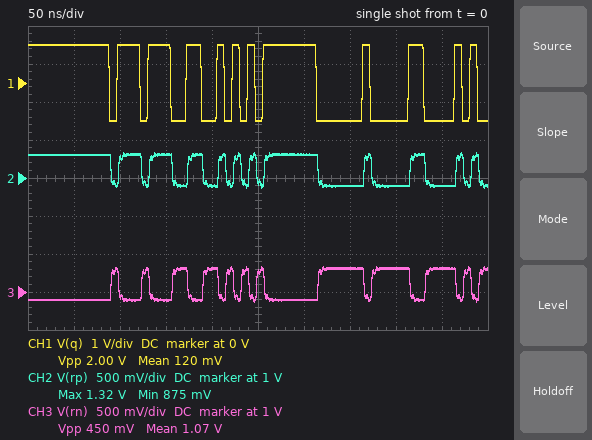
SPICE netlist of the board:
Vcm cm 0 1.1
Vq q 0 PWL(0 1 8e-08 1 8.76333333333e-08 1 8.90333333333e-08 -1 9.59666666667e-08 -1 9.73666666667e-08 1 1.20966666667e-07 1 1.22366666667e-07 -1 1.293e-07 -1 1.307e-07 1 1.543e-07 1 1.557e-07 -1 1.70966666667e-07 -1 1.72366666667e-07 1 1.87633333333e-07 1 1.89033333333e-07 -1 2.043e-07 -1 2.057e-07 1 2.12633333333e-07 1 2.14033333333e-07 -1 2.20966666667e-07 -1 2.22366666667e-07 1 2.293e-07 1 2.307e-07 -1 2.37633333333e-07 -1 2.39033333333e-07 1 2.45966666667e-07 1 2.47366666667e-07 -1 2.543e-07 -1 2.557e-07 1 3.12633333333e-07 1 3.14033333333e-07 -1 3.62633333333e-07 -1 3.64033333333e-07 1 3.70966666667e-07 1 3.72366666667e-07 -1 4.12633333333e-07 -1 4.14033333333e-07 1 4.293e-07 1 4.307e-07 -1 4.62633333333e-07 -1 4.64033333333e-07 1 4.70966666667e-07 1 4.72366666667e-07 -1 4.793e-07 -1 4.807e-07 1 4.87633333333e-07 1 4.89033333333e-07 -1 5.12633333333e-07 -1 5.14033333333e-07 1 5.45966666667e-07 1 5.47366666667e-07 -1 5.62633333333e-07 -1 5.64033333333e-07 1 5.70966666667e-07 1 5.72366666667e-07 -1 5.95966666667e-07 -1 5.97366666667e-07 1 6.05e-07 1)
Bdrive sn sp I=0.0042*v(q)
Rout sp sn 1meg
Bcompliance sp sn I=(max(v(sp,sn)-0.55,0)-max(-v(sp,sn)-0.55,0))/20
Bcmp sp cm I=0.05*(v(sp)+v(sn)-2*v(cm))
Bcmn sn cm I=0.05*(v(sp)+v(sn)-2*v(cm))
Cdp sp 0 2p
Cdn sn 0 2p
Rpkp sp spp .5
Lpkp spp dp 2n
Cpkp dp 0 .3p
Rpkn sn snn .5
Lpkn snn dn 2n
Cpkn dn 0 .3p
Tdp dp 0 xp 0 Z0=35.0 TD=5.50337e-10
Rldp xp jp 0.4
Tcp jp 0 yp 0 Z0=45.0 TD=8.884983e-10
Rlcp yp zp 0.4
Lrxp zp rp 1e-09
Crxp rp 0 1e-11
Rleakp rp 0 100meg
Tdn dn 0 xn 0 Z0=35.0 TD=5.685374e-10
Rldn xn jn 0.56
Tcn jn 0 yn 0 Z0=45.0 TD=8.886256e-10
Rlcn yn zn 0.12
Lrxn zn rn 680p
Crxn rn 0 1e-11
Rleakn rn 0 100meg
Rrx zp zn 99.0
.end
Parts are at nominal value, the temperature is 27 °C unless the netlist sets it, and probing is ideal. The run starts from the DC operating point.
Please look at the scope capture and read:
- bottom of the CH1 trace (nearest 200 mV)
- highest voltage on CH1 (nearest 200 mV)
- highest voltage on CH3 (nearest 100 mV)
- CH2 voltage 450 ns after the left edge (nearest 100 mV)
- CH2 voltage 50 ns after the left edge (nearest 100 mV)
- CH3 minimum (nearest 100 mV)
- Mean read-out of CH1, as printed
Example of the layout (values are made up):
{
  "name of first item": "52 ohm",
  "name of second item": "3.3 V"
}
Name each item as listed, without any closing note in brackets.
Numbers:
{
  "bottom of the CH1 trace": "-1.0 V",
  "highest voltage on CH1": "1.0 V",
  "highest voltage on CH3": "1.3 V",
  "CH2 voltage 450 ns after the left edge": "900 mV",
  "CH2 voltage 50 ns after the left edge": "1.3 V",
  "CH3 minimum": "900 mV",
  "Mean read-out of CH1, as printed": "120 mV"
}
